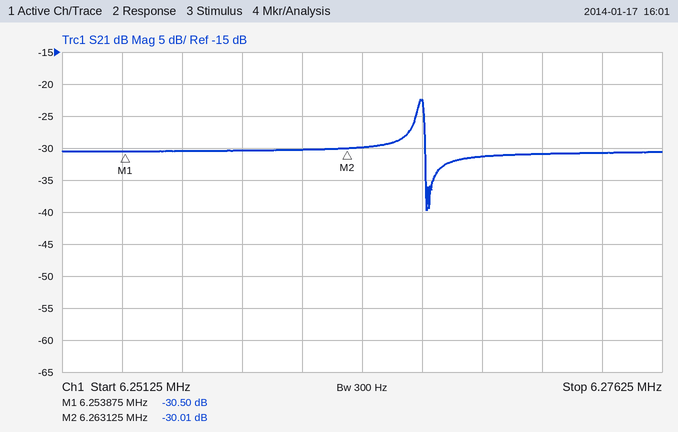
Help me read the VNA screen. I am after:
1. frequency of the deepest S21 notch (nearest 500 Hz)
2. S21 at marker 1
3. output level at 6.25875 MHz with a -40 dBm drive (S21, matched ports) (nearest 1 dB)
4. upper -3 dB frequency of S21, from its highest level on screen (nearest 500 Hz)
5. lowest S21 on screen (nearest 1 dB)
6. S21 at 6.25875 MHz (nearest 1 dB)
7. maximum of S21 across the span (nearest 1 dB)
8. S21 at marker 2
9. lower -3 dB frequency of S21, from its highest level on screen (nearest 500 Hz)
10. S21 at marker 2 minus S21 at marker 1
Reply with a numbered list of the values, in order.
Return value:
1. 6.2665 MHz
2. -30.50 dB
3. -70 dBm
4. 6.2665 MHz
5. -40 dB
6. -30 dB
7. -22 dB
8. -30.01 dB
9. 6.2660 MHz
10. 0.49 dB
